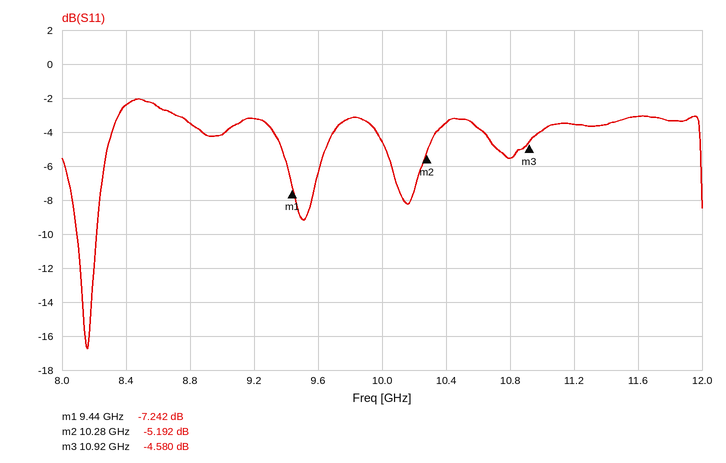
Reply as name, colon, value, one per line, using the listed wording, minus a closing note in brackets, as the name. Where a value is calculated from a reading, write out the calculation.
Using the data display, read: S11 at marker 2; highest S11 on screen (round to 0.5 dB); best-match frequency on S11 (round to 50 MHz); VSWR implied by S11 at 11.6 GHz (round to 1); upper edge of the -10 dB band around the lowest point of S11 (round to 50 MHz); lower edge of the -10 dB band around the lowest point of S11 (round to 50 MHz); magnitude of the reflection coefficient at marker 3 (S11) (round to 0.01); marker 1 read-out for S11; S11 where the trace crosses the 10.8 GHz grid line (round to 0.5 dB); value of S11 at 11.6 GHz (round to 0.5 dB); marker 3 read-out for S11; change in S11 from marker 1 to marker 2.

S11 at marker 2: -5.192 dB
highest S11 on screen: -2.0 dB
best-match frequency on S11: 8.15 GHz
VSWR implied by S11 at 11.6 GHz: |Γ| = 10^(-3/20) = 0.7079; VSWR = (1 + 0.7079)/(1 − 0.7079) ≈ 6
upper edge of the -10 dB band around the lowest point of S11: 8.20 GHz
lower edge of the -10 dB band around the lowest point of S11: 8.10 GHz
magnitude of the reflection coefficient at marker 3 (S11): 10^(-4.58/20) ≈ 0.59
marker 1 read-out for S11: -7.242 dB
S11 where the trace crosses the 10.8 GHz grid line: -5.5 dB
value of S11 at 11.6 GHz: -3.0 dB
marker 3 read-out for S11: -4.580 dB
change in S11 from marker 1 to marker 2: -5.192 − (-7.242) = 2.050 dB
